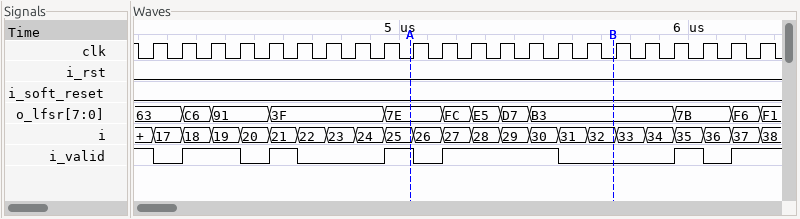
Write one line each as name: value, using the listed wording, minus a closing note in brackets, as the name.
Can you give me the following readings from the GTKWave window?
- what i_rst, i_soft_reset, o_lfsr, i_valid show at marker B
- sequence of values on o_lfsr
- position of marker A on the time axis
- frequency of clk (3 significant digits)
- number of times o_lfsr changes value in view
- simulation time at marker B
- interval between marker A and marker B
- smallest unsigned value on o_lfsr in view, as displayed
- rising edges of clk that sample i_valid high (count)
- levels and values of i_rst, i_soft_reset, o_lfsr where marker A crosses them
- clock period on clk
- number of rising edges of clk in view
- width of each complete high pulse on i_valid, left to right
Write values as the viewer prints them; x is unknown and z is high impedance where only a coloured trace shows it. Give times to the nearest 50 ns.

what i_rst, i_soft_reset, o_lfsr, i_valid show at marker B: i_rst=0, i_soft_reset=0, o_lfsr=B3, i_valid=0
sequence of values on o_lfsr: 63, C6, 91, 3F, 7E, FC, E5, D7, B3, 7B, F6, F1
position of marker A on the time axis: 5050 ns
frequency of clk: 10.0 MHz
number of times o_lfsr changes value in view: 11
simulation time at marker B: 5750 ns
interval between marker A and marker B: 700 ns
smallest unsigned value on o_lfsr in view, as displayed: 3F
rising edges of clk that sample i_valid high: 11
levels and values of i_rst, i_soft_reset, o_lfsr where marker A crosses them: i_rst=0, i_soft_reset=0, o_lfsr=7E
clock period on clk: 100 ns
number of rising edges of clk in view: 22
width of each complete high pulse on i_valid, left to right: 200 ns, 100 ns, 100 ns, 400 ns, 100 ns
